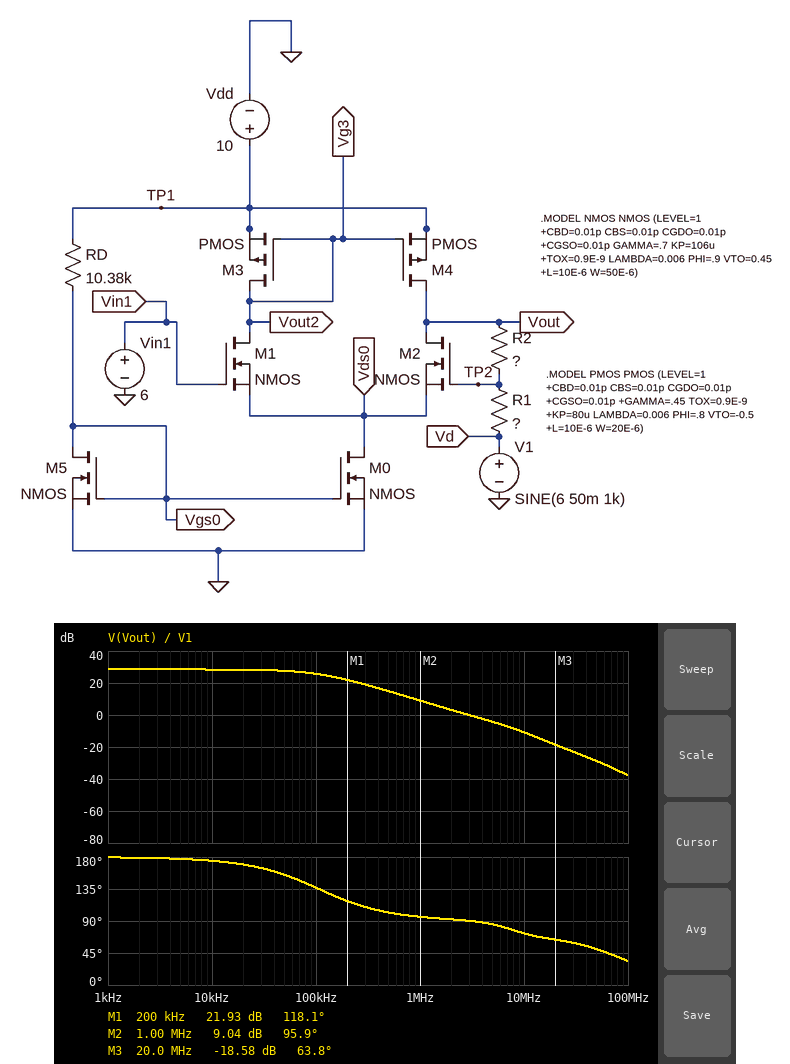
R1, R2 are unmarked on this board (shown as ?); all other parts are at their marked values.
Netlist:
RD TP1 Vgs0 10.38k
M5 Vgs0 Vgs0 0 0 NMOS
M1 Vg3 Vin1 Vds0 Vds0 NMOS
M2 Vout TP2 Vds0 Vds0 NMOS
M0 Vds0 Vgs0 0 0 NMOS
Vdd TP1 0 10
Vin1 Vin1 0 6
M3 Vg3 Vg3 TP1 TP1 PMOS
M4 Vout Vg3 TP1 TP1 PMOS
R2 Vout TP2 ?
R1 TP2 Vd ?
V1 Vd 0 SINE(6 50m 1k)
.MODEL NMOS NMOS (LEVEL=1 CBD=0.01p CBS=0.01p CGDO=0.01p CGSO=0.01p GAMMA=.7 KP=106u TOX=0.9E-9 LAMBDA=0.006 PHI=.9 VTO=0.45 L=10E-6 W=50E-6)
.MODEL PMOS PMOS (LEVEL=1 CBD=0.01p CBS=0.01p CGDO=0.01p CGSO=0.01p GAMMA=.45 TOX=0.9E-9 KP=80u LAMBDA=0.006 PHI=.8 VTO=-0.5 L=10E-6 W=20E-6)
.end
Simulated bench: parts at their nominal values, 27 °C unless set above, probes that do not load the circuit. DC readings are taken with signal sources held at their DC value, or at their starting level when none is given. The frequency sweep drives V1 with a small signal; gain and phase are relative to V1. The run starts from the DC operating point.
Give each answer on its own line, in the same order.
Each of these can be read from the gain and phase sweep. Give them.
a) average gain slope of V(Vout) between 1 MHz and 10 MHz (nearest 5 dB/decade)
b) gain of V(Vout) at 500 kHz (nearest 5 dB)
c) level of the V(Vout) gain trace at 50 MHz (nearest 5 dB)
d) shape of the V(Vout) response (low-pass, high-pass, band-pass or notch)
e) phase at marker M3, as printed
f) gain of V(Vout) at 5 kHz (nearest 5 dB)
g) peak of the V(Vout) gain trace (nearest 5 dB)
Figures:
-20 dB/decade
15 dB
-30 dB
low-pass
63.8 deg
30 dB
30 dB
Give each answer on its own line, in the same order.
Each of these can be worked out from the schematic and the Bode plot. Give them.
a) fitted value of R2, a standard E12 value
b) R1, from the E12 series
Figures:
27 MΩ
820 kΩ
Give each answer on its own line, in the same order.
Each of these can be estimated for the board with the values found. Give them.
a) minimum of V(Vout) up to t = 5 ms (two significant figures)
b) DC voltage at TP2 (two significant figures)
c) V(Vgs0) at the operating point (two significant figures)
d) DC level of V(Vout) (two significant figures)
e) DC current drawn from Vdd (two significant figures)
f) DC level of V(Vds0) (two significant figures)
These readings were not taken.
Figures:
5.4 V
6.0 V
2.1 V
6.3 V
1.5 mA
4.4 V
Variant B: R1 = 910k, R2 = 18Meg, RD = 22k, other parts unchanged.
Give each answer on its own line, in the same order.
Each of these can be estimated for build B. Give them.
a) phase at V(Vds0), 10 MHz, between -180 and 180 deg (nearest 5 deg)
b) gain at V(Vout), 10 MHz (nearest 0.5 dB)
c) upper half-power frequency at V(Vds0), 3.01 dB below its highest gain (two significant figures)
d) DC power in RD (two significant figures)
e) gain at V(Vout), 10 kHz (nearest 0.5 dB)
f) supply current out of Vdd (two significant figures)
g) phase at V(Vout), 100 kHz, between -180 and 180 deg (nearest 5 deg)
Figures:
-70 deg
-10.0 dB
200 kHz
3.2 mW
25.0 dB
770 µA
155 deg
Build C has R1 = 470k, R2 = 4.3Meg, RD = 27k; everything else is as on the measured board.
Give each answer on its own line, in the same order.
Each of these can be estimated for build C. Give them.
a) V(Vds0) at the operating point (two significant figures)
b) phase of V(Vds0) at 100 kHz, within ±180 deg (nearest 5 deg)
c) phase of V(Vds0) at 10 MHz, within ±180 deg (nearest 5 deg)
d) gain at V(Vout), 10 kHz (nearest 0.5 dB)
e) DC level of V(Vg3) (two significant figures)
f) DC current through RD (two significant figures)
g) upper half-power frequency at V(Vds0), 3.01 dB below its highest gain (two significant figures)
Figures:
4.8 V
-5 deg
-70 deg
19.0 dB
8.1 V
310 µA
940 kHz
